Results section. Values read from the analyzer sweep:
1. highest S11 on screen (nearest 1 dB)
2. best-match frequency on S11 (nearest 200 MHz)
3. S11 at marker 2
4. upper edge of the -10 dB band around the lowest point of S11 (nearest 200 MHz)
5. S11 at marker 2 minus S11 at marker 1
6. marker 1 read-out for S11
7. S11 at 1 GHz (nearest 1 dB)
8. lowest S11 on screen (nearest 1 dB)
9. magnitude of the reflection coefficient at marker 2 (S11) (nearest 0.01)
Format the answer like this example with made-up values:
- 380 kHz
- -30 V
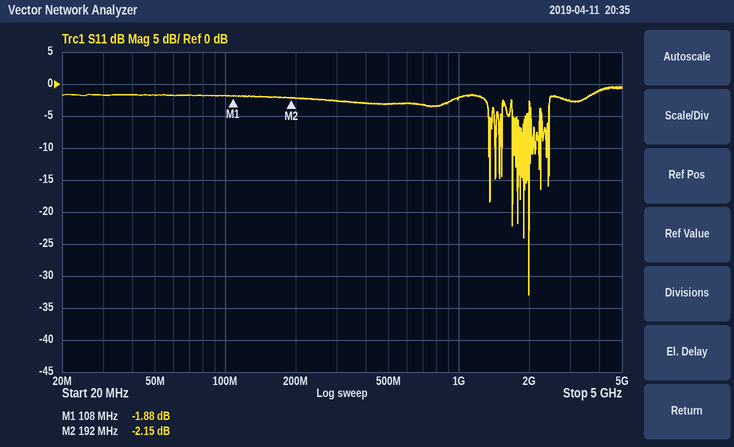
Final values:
- 0 dB
- 2.0 GHz
- -2.15 dB
- 2.0 GHz
- -0.27 dB
- -1.88 dB
- -2 dB
- -33 dB
- 0.78
